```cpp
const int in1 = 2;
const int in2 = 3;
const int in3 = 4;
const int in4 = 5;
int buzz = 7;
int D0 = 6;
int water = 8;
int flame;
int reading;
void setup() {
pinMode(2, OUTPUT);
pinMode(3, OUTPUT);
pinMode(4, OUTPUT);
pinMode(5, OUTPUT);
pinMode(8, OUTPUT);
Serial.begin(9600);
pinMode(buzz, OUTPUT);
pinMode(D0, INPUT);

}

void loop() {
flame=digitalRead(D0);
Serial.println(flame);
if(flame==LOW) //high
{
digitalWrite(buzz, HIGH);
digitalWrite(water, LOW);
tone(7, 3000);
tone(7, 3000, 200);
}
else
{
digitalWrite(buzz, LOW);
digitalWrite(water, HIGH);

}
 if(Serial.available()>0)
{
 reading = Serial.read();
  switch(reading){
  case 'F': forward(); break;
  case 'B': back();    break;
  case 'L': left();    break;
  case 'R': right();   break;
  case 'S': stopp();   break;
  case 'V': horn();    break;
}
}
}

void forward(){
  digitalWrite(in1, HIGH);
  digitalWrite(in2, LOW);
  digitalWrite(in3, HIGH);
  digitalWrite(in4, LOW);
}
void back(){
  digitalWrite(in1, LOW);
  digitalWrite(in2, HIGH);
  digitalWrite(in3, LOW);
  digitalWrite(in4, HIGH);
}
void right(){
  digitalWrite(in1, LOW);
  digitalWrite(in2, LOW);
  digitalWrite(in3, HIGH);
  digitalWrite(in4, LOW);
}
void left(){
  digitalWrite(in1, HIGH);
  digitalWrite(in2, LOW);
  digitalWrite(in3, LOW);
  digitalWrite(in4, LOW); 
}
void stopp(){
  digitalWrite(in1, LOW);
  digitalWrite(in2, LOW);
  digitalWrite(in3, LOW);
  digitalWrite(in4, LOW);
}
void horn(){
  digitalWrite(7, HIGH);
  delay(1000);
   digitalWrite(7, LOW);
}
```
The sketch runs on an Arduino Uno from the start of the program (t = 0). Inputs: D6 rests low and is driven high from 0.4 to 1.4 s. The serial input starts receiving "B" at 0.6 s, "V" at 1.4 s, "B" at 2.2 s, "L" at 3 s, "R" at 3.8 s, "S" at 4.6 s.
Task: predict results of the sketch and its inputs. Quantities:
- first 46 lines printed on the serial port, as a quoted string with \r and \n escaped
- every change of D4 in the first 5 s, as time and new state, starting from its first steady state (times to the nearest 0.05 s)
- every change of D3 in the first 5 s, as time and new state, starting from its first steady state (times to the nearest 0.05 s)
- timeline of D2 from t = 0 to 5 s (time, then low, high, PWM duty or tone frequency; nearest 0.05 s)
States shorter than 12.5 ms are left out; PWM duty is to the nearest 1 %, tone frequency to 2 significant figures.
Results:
"0\r\n0\r\n0\r\n0\r\n0\r\n0\r\n0\r\n0\r\n0\r\n0\r\n0\r\n0\r\n0\r\n0\r\n0\r\n0\r\n0\r\n0\r\n0\r\n0\r\n0\r\n0\r\n0\r\n0\r\n0\r\n0\r\n0\r\n0\r\n0\r\n0\r\n0\r\n0\r\n0\r\n0\r\n0\r\n0\r\n0\r\n0\r\n0\r\n0\r\n0\r\n0\r\n0\r\n0\r\n0\r\n0\r\n"
0 s low; 3.8 s high; 4.6 s low
0 s low; 0.6 s high; 3 s low
0 s low; 3 s high; 3.8 s low
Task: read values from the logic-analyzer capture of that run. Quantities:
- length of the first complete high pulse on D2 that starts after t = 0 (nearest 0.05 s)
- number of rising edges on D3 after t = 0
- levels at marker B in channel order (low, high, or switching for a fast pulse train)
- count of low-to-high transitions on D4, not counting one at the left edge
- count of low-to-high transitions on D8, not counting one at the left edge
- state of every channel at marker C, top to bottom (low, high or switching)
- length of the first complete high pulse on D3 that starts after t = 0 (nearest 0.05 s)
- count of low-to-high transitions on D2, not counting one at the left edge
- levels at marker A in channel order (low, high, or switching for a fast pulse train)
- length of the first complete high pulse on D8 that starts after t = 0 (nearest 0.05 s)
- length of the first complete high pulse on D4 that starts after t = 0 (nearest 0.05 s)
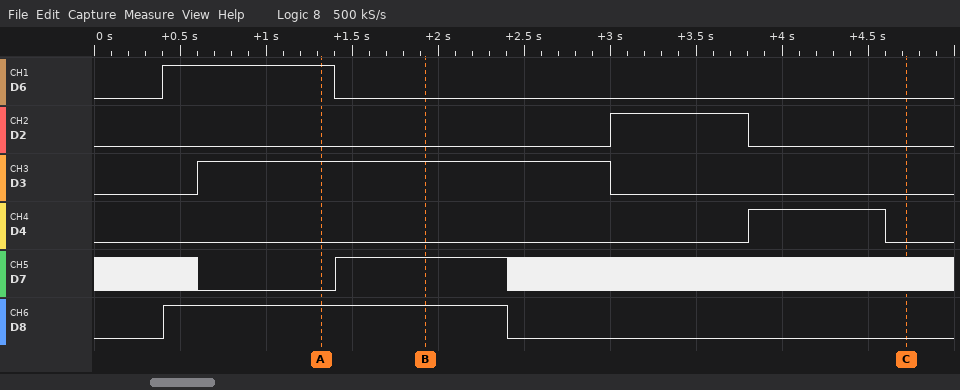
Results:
0.80 s
1
D6 low, D2 low, D3 high, D4 low, D7 high, D8 high
1
1
D6 low, D2 low, D3 low, D4 low, D7 switching, D8 low
2.40 s
1
D6 high, D2 low, D3 high, D4 low, D7 low, D8 high
2.00 s
0.80 s
